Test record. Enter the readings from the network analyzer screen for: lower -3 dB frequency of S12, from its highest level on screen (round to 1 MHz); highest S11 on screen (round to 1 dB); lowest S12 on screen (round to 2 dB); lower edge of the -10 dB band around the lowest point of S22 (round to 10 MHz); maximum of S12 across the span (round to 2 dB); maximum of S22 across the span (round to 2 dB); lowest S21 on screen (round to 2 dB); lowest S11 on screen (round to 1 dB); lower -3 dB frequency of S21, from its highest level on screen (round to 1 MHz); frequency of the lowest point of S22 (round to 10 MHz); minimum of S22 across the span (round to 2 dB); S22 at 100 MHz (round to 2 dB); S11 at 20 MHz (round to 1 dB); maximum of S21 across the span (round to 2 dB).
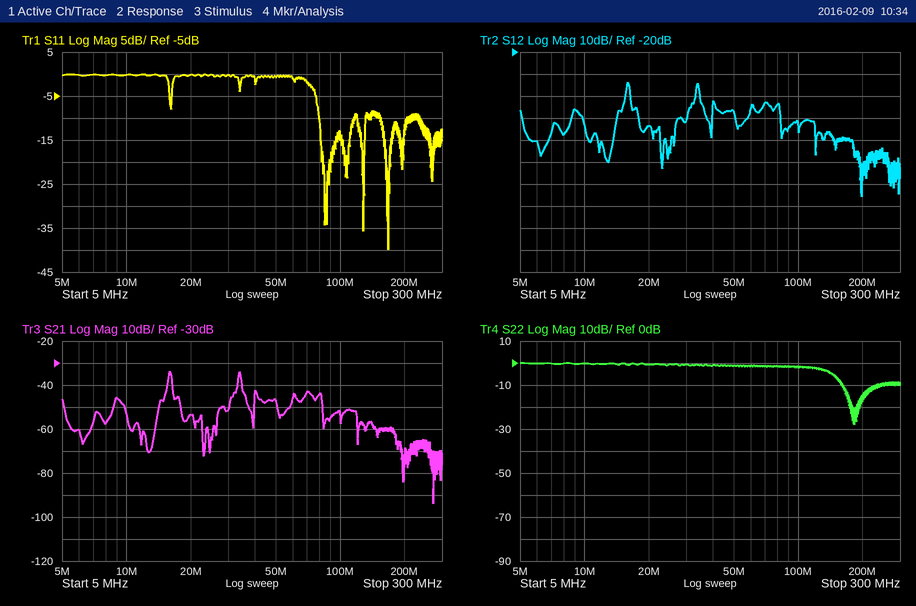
16 MHz
0 dB
-86 dB
160 MHz
-34 dB
0 dB
-94 dB
-40 dB
16 MHz
180 MHz
-28 dB
-2 dB
0 dB
-34 dB
